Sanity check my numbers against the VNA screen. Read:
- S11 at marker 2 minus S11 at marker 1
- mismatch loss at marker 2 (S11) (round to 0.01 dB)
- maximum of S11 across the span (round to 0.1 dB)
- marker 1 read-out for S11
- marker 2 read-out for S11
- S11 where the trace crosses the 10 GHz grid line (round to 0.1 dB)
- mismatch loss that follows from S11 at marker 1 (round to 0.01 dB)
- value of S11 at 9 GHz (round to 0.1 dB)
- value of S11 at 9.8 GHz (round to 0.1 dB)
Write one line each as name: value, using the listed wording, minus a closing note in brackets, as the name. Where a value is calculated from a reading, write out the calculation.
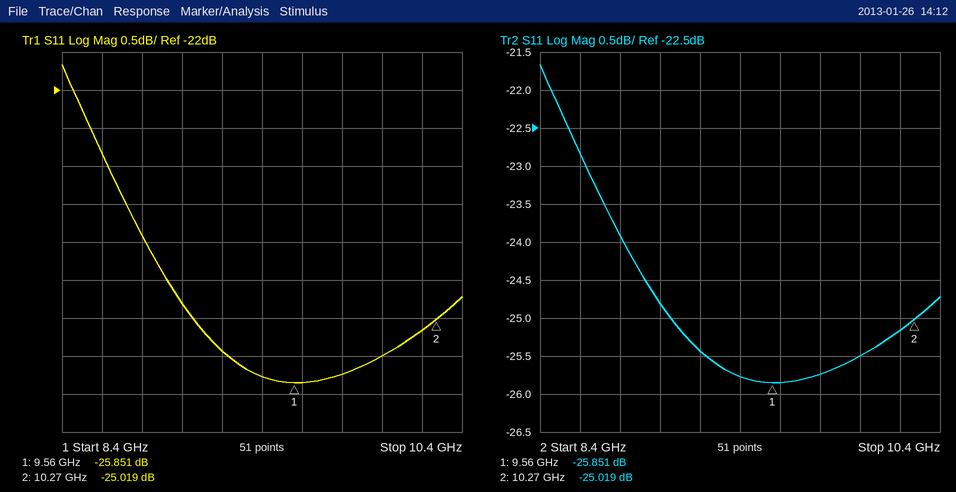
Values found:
S11 at marker 2 minus S11 at marker 1: -25.019 − (-25.851) = 0.832 dB
mismatch loss at marker 2 (S11): −10 log10(1 − 10^(-25.019/10)) ≈ 0.01 dB
maximum of S11 across the span: -21.7 dB
marker 1 read-out for S11: -25.851 dB
marker 2 read-out for S11: -25.019 dB
S11 where the trace crosses the 10 GHz grid line: -25.5 dB
mismatch loss that follows from S11 at marker 1: −10 log10(1 − 10^(-25.851/10)) ≈ 0.01 dB
value of S11 at 9 GHz: -24.8 dB
value of S11 at 9.8 GHz: -25.7 dB
